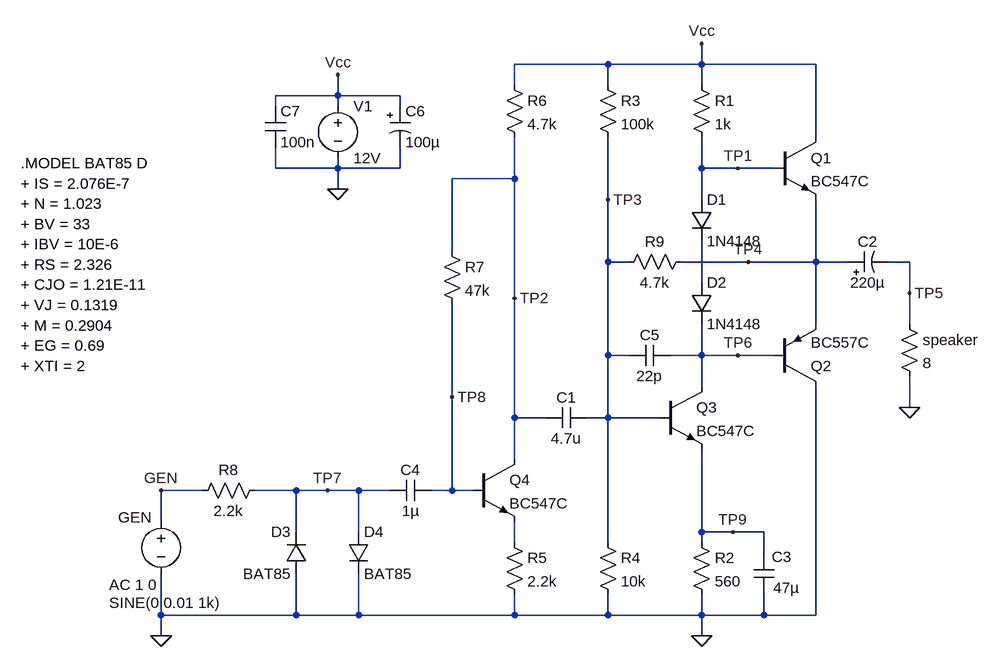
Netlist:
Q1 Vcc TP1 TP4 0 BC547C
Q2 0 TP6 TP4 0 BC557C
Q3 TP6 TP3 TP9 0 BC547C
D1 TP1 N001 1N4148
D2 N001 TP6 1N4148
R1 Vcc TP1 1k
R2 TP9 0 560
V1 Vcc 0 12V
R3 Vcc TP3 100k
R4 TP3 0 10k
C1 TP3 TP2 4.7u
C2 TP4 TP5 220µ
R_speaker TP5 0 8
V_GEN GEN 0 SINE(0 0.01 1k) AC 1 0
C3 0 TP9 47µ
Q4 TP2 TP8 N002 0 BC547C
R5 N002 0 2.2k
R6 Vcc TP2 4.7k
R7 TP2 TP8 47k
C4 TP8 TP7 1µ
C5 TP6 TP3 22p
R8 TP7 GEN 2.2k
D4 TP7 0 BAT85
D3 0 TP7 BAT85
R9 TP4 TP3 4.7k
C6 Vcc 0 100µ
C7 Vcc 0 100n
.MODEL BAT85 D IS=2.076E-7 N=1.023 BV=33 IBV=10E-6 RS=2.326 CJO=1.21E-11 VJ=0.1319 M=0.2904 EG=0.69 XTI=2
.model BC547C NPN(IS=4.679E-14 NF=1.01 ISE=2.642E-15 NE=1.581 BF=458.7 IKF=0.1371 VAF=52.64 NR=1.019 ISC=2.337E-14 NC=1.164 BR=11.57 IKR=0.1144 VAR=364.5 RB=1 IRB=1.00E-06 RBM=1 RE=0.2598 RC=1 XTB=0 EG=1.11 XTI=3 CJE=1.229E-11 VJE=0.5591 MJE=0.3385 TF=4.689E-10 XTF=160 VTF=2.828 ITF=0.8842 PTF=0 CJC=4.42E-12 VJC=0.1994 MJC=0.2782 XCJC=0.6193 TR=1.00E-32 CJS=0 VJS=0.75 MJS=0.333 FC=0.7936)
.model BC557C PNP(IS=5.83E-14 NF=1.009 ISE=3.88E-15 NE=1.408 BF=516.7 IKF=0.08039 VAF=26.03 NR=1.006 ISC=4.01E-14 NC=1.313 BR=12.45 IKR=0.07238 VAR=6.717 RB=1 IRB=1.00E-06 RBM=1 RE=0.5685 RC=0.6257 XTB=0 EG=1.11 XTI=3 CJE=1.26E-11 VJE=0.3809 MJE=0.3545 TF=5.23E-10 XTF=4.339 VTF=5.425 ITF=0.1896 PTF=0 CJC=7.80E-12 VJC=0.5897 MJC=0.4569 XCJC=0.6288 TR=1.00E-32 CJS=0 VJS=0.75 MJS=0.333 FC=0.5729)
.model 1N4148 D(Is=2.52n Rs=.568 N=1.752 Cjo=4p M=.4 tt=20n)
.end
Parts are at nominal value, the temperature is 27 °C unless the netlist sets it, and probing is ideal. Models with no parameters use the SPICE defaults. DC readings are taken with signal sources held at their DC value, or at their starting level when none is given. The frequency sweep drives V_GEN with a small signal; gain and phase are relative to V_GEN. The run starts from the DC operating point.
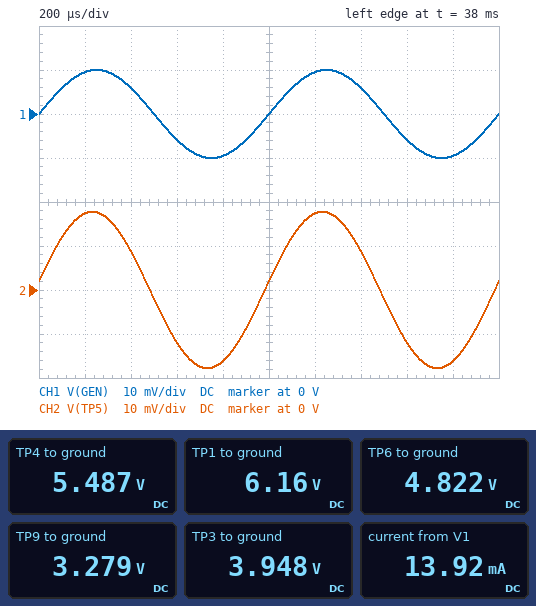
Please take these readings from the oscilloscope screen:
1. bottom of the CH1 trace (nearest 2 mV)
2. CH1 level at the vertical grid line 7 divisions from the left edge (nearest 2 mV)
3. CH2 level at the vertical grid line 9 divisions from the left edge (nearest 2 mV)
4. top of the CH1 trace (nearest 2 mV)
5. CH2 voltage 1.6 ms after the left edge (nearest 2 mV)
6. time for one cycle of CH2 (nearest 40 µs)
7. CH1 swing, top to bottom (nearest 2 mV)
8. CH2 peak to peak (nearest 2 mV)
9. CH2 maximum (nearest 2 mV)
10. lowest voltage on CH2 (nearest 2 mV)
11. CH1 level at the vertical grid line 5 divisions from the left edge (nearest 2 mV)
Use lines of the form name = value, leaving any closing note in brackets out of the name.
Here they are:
bottom of the CH1 trace = -10 mV
CH1 level at the vertical grid line 7 divisions from the left edge = 6 mV
CH2 level at the vertical grid line 9 divisions from the left edge = -16 mV
top of the CH1 trace = 10 mV
CH2 voltage 1.6 ms after the left edge = -12 mV
time for one cycle of CH2 = 1.00 ms
CH1 swing, top to bottom = 20 mV
CH2 peak to peak = 36 mV
CH2 maximum = 18 mV
lowest voltage on CH2 = -18 mV
CH1 level at the vertical grid line 5 divisions from the left edge = 0 V
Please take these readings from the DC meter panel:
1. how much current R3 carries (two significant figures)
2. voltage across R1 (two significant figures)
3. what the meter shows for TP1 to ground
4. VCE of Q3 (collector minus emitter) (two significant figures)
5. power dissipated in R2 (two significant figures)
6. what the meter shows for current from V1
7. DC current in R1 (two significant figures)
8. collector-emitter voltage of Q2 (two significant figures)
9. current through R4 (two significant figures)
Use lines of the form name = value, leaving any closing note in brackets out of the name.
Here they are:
how much current R3 carries = 81 µA
voltage across R1 = 5.8 V
what the meter shows for TP1 to ground = 6.16 V
VCE of Q3 (collector minus emitter) = 1.5 V
power dissipated in R2 = 19 mW
what the meter shows for current from V1 = 13.92 mA
DC current in R1 = 5.8 mA
collector-emitter voltage of Q2 = -5.5 V
current through R4 = 390 µA
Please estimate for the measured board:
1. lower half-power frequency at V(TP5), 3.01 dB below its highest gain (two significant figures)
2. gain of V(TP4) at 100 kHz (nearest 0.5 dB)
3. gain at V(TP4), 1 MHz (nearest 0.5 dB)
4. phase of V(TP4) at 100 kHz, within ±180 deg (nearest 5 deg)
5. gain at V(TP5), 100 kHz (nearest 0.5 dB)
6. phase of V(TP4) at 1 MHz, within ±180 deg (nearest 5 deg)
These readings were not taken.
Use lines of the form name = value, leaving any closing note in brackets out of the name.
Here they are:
lower half-power frequency at V(TP5), 3.01 dB below its highest gain = 97 Hz
gain of V(TP4) at 100 kHz = 5.0 dB
gain at V(TP4), 1 MHz = 1.5 dB
phase of V(TP4) at 100 kHz, within ±180 deg = -10 deg
gain at V(TP5), 100 kHz = 5.0 dB
phase of V(TP4) at 1 MHz, within ±180 deg = -70 deg
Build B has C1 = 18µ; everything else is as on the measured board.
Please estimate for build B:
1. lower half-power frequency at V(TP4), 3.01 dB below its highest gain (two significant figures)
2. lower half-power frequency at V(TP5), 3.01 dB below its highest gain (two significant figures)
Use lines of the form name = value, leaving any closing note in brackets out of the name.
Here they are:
lower half-power frequency at V(TP4), 3.01 dB below its highest gain = 13 Hz
lower half-power frequency at V(TP5), 3.01 dB below its highest gain = 96 Hz
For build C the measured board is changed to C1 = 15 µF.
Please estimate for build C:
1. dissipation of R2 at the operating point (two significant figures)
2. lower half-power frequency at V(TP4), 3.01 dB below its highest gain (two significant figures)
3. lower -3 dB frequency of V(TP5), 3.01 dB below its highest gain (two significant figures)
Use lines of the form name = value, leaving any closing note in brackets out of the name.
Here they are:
dissipation of R2 at the operating point = 19 mW
lower half-power frequency at V(TP4), 3.01 dB below its highest gain = 13 Hz
lower -3 dB frequency of V(TP5), 3.01 dB below its highest gain = 96 Hz
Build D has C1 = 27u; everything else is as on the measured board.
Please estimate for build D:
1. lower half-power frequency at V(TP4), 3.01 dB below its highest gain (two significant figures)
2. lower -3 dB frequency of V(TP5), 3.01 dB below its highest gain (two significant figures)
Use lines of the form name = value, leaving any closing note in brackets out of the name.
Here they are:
lower half-power frequency at V(TP4), 3.01 dB below its highest gain = 13 Hz
lower -3 dB frequency of V(TP5), 3.01 dB below its highest gain = 96 Hz
